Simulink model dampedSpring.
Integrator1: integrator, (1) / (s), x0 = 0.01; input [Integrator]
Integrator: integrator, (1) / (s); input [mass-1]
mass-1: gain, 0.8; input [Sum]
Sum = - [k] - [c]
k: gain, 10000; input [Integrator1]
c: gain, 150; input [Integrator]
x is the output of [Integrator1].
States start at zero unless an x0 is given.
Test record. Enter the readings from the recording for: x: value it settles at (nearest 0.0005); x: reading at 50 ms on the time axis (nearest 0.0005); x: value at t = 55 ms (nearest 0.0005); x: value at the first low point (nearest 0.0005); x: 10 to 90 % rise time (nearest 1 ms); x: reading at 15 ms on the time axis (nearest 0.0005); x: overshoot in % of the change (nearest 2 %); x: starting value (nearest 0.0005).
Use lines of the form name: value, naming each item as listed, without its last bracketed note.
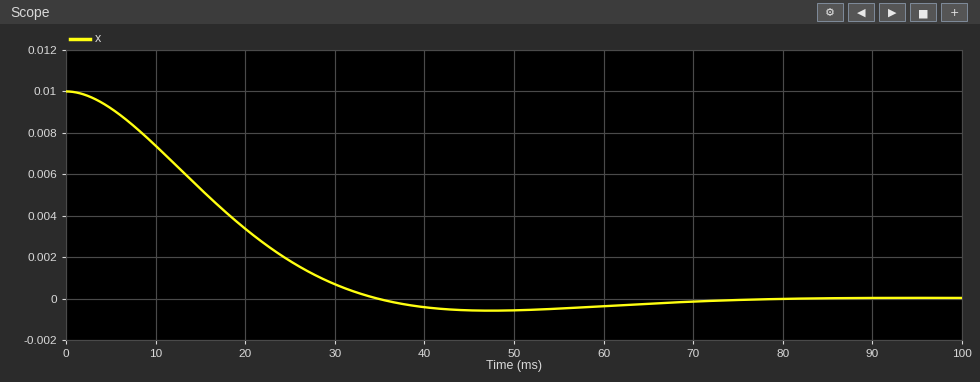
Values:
x: value it settles at: 0.0000
x: reading at 50 ms on the time axis: -0.0005
x: value at t = 55 ms: -0.0005
x: value at the first low point: -0.0005
x: 10 to 90 % rise time: 23 ms
x: reading at 15 ms on the time axis: 0.0055
x: overshoot in % of the change: 6 %
x: starting value: 0.0100
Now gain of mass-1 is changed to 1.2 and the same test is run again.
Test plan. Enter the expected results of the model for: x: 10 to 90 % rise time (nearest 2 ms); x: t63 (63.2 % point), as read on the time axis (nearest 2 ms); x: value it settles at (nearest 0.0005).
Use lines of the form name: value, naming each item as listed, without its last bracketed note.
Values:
x: 10 to 90 % rise time: 24 ms
x: t63 (63.2 % point), as read on the time axis: 18 ms
x: value it settles at: 0.0000
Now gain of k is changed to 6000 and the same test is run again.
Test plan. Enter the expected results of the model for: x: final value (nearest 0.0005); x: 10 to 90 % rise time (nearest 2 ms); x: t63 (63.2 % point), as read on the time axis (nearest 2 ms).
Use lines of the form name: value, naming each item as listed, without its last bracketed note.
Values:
x: final value: 0.0000
x: 10 to 90 % rise time: 40 ms
x: t63 (63.2 % point), as read on the time axis: 28 ms
